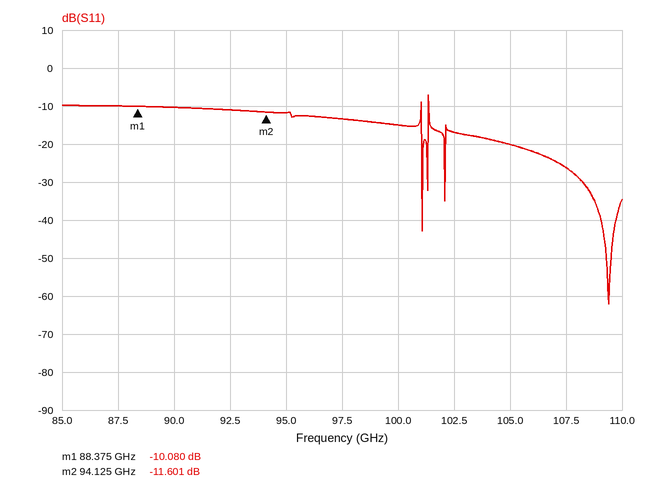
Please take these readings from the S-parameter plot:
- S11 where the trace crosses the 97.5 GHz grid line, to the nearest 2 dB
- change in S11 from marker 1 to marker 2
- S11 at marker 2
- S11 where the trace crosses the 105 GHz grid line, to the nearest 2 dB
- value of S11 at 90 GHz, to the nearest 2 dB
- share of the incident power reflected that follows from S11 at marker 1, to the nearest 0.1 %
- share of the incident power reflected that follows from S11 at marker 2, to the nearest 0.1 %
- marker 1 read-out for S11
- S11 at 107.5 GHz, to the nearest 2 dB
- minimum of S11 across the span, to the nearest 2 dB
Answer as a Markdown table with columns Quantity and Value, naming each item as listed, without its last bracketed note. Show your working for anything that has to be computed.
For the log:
| Quantity | Value |
|---|---|
| S11 where the trace crosses the 97.5 GHz grid line, to the nearest 2 dB | -14 dB |
| change in S11 from marker 1 to marker 2 | -11.601 − (-10.08) = -1.521 dB |
| S11 at marker 2 | -11.601 dB |
| S11 where the trace crosses the 105 GHz grid line, to the nearest 2 dB | -20 dB |
| value of S11 at 90 GHz, to the nearest 2 dB | -10 dB |
| share of the incident power reflected that follows from S11 at marker 1, to the nearest 0.1 % | 10^(-10.08/10) ≈ 9.8 % |
| share of the incident power reflected that follows from S11 at marker 2, to the nearest 0.1 % | 10^(-11.601/10) ≈ 6.9 % |
| marker 1 read-out for S11 | -10.080 dB |
| S11 at 107.5 GHz, to the nearest 2 dB | -26 dB |
| minimum of S11 across the span, to the nearest 2 dB | -62 dB |
